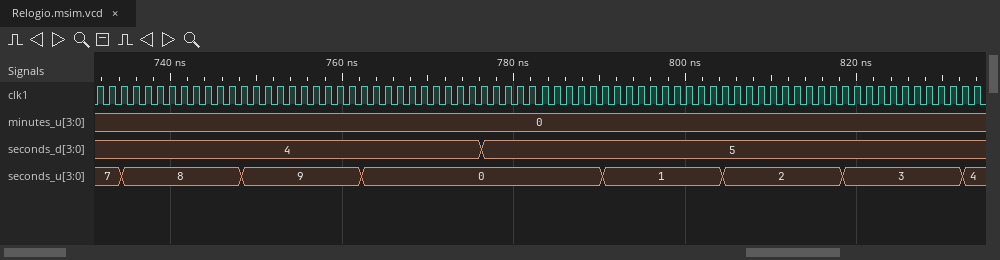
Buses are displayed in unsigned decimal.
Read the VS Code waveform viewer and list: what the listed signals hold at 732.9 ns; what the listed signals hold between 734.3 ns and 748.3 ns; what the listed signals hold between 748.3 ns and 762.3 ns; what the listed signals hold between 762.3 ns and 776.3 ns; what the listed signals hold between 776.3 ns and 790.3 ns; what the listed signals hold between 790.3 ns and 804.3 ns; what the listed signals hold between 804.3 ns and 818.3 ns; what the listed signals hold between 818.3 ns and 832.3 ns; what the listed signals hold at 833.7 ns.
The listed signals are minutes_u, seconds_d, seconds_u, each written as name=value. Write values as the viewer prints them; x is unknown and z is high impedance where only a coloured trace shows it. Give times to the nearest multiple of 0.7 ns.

minutes_u=0, seconds_d=4, seconds_u=7
minutes_u=0, seconds_d=4, seconds_u=8
minutes_u=0, seconds_d=4, seconds_u=9
minutes_u=0, seconds_d=4, seconds_u=0
minutes_u=0, seconds_d=5, seconds_u=0
minutes_u=0, seconds_d=5, seconds_u=1
minutes_u=0, seconds_d=5, seconds_u=2
minutes_u=0, seconds_d=5, seconds_u=3
minutes_u=0, seconds_d=5, seconds_u=4
